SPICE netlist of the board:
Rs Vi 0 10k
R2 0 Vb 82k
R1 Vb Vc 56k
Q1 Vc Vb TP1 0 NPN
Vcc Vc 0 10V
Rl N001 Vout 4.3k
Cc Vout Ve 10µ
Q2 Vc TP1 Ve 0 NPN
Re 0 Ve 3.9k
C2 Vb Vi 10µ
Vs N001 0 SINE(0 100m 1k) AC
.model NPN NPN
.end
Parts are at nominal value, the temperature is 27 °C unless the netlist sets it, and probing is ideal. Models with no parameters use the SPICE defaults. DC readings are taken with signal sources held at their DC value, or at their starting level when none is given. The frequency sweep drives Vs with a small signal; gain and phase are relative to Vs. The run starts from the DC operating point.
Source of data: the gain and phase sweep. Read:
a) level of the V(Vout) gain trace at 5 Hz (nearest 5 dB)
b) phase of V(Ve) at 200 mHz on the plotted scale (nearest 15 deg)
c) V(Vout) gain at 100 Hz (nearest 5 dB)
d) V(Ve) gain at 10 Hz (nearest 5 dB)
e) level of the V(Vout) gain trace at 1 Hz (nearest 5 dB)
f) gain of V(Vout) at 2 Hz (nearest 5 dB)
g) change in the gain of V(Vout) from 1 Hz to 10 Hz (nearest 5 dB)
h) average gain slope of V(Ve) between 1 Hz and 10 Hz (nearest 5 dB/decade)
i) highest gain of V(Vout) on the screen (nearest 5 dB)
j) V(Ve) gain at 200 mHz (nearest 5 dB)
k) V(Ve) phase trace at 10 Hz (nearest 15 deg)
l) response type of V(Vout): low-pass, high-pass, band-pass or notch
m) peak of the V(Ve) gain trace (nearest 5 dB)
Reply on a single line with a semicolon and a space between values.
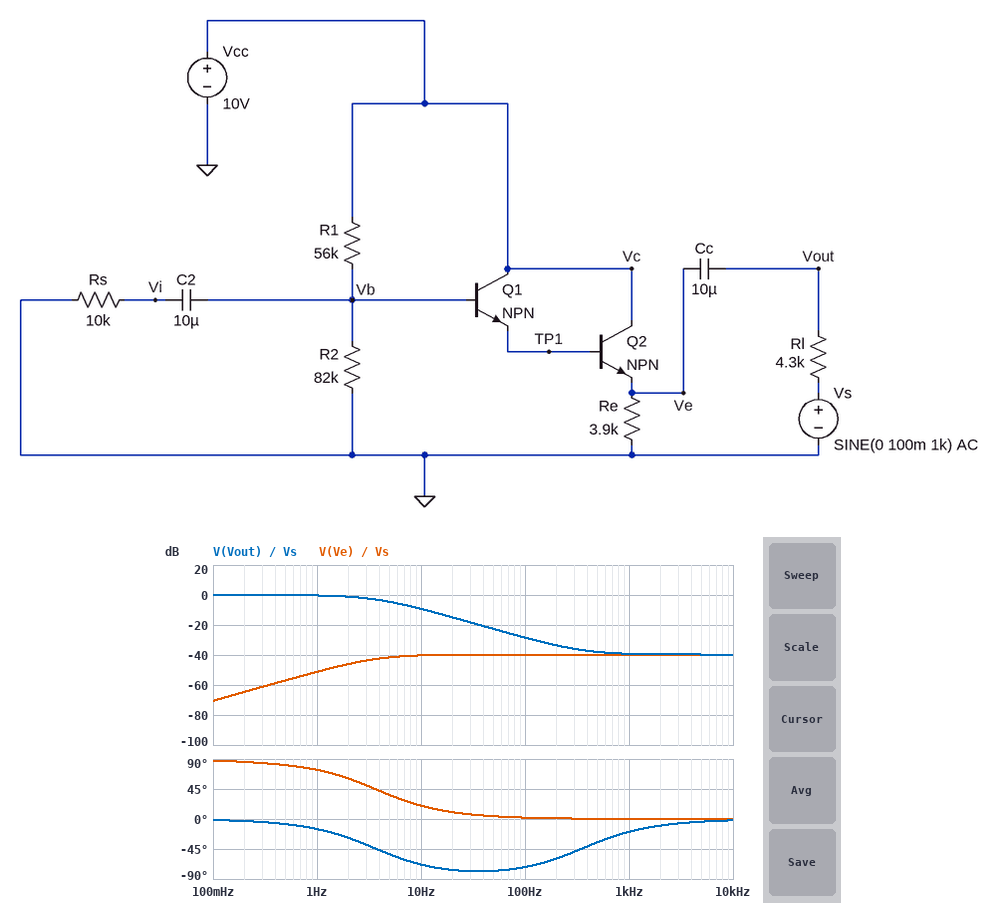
-5 dB; 90 deg; -30 dB; -40 dB; 0 dB; 0 dB; -10 dB; 10 dB/decade; 0 dB; -65 dB; 15 deg; low-pass; -40 dB
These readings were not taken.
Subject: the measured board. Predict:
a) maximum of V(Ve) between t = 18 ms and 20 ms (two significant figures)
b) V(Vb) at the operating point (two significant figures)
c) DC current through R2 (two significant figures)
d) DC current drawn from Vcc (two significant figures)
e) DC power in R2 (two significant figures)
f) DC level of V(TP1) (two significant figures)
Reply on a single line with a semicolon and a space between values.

4.5 V; 5.9 V; 72 µA; 1.2 mA; 430 µW; 5.3 V
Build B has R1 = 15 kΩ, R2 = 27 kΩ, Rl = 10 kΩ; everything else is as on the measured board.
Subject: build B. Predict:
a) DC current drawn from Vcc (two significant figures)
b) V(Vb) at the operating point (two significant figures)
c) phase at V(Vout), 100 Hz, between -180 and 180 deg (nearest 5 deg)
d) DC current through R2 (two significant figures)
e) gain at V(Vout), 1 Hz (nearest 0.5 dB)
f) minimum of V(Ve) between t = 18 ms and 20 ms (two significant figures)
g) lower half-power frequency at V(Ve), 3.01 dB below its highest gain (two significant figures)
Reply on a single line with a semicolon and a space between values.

1.5 mA; 6.4 V; -75 deg; 240 µA; -1.5 dB; 5.0 V; 1.6 Hz
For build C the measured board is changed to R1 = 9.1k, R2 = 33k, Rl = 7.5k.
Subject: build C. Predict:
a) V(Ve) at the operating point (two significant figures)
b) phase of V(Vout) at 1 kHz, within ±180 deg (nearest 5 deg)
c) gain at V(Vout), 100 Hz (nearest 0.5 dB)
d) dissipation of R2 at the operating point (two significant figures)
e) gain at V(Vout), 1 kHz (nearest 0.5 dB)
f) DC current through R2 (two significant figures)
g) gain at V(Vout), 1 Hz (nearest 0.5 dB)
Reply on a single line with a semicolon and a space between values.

6.4 V; -25 deg; -33.5 dB; 1.9 mW; -46.5 dB; 240 µA; -1.0 dB
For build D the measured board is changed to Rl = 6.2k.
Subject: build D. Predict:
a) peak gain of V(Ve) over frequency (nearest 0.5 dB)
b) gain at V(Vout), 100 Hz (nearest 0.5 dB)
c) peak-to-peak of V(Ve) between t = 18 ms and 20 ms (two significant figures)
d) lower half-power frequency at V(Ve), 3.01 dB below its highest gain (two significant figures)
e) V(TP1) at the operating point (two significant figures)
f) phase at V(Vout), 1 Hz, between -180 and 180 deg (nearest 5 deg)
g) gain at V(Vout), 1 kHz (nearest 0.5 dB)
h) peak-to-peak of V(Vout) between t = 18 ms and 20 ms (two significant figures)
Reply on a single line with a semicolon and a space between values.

-43.0 dB; -31.5 dB; 1.4 mV; 2.5 Hz; 5.3 V; -20 deg; -42.5 dB; 1.5 mV
